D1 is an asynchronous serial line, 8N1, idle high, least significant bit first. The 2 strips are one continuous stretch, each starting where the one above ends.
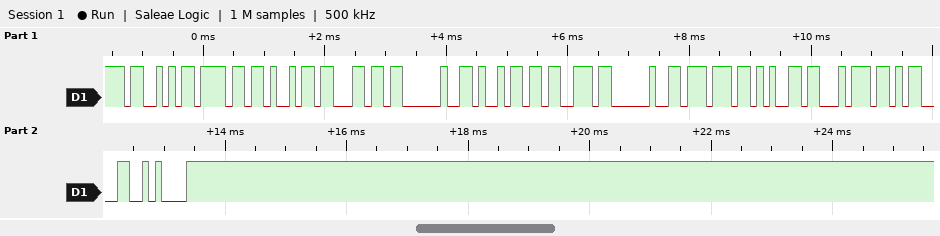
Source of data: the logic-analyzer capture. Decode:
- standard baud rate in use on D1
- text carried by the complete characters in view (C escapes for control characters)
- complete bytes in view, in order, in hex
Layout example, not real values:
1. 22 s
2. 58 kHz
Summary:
1. 9600 baud
2. "Soil is wet\r\n"
3. 0x53 0x6F 0x69 0x6C 0x20 0x69 0x73 0x20 0x77 0x65 0x74 0x0D 0x0A
